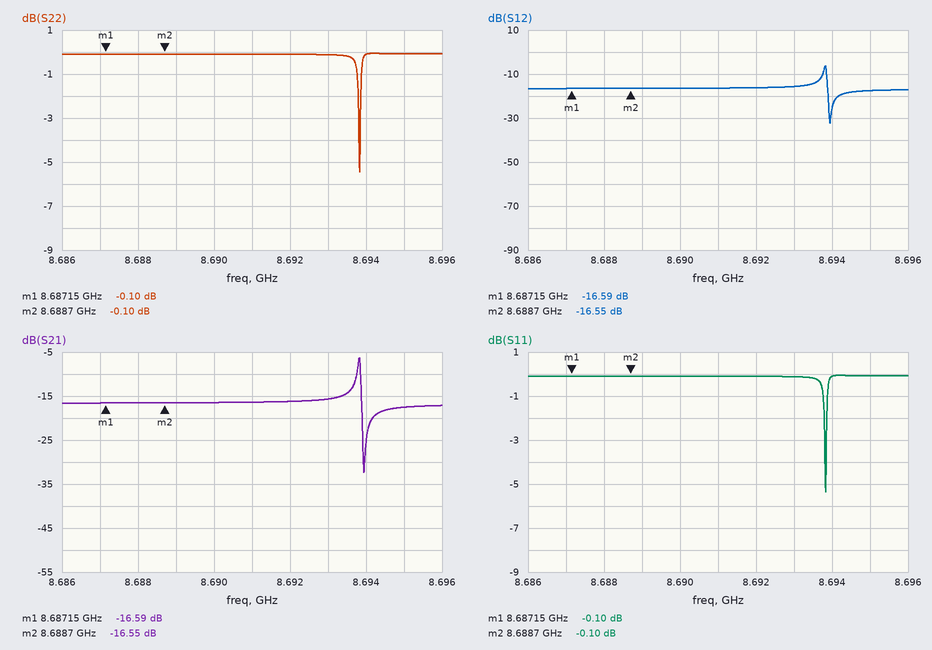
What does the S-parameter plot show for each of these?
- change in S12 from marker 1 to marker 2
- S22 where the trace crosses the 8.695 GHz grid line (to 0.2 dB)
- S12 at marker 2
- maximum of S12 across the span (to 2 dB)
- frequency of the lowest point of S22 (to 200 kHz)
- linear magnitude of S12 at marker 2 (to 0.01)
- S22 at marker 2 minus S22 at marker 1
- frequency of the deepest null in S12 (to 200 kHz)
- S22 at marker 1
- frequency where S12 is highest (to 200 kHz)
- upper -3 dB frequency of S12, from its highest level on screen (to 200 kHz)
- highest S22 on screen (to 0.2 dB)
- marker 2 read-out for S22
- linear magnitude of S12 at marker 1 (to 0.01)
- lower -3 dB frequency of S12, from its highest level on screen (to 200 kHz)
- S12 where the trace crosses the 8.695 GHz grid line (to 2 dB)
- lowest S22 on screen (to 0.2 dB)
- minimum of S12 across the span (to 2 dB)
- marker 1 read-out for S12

0.04 dB
0.0 dB
-16.55 dB
-6 dB
8.6938 GHz
0.15
0.00 dB
8.6940 GHz
-0.10 dB
8.6938 GHz
8.6938 GHz
0.0 dB
-0.10 dB
0.15
8.6938 GHz
-18 dB
-5.4 dB
-32 dB
-16.59 dB
